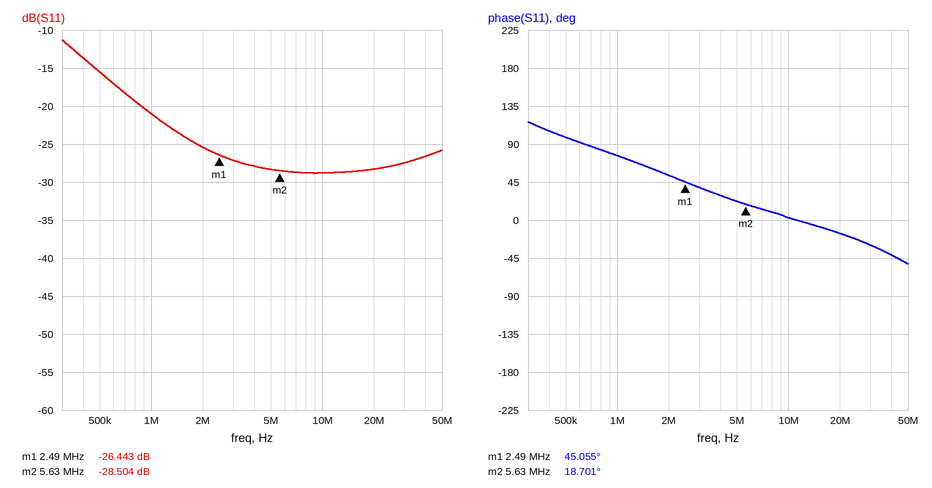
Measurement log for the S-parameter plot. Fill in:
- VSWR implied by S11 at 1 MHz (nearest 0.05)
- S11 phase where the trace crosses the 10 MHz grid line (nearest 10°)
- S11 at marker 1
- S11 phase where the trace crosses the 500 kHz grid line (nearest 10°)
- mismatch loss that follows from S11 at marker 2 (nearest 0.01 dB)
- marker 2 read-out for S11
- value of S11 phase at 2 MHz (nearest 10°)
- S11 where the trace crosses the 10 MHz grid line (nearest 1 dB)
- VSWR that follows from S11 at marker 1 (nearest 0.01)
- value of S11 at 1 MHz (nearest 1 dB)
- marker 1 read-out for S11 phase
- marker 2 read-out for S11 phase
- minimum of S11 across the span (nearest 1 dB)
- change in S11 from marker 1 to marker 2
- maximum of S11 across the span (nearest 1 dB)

1.20
0°
-26.443 dB
100°
0.01 dB
-28.504 dB
50°
-29 dB
1.10
-21 dB
45.055°
18.701°
-29 dB
-2.061 dB
-11 dB
